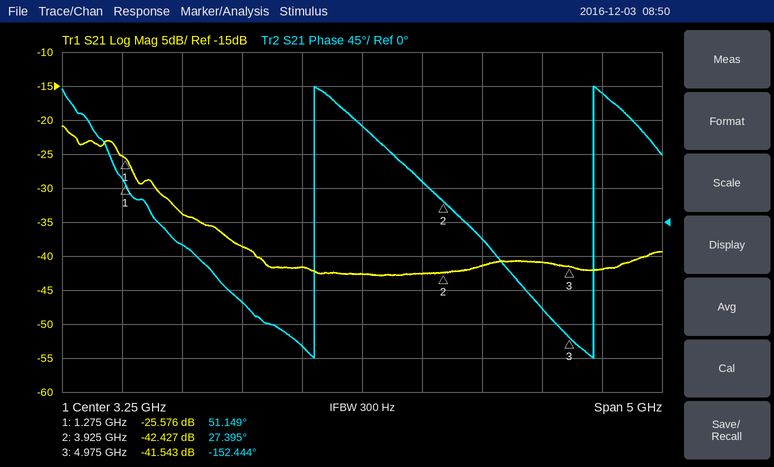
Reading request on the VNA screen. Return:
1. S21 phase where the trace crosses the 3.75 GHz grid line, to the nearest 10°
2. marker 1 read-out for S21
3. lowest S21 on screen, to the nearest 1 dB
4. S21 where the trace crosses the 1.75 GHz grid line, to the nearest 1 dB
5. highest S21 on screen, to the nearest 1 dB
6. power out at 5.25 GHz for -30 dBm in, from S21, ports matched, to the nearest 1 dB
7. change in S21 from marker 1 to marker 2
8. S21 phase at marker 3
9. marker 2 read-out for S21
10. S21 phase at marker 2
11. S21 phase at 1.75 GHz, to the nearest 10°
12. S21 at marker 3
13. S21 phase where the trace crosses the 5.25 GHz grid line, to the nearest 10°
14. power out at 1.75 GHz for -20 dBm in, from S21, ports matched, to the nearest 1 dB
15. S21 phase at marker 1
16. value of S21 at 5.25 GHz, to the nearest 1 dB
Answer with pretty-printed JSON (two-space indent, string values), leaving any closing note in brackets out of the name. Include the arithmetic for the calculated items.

{
  "S21 phase where the trace crosses the 3.75 GHz grid line, to the nearest 10°": "50°",
  "marker 1 read-out for S21": "-25.576 dB",
  "lowest S21 on screen, to the nearest 1 dB": "-43 dB",
  "S21 where the trace crosses the 1.75 GHz grid line, to the nearest 1 dB": "-34 dB",
  "highest S21 on screen, to the nearest 1 dB": "-21 dB",
  "power out at 5.25 GHz for -30 dBm in, from S21, ports matched, to the nearest 1 dB": "-30 dBm + (-42 dB) = -72 dBm",
  "change in S21 from marker 1 to marker 2": "-42.427 − (-25.576) = -16.851 dB",
  "S21 phase at marker 3": "-152.444°",
  "marker 2 read-out for S21": "-42.427 dB",
  "S21 phase at marker 2": "27.395°",
  "S21 phase at 1.75 GHz, to the nearest 10°": "-30°",
  "S21 at marker 3": "-41.543 dB",
  "S21 phase where the trace crosses the 5.25 GHz grid line, to the nearest 10°": "170°",
  "power out at 1.75 GHz for -20 dBm in, from S21, ports matched, to the nearest 1 dB": "-20 dBm + (-34 dB) = -54 dBm",
  "S21 phase at marker 1": "51.149°",
  "value of S21 at 5.25 GHz, to the nearest 1 dB": "-42 dB"
}
